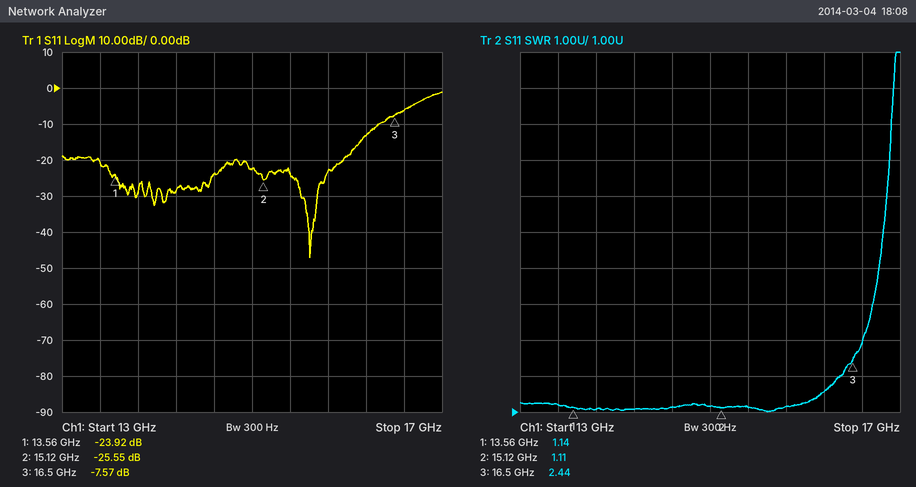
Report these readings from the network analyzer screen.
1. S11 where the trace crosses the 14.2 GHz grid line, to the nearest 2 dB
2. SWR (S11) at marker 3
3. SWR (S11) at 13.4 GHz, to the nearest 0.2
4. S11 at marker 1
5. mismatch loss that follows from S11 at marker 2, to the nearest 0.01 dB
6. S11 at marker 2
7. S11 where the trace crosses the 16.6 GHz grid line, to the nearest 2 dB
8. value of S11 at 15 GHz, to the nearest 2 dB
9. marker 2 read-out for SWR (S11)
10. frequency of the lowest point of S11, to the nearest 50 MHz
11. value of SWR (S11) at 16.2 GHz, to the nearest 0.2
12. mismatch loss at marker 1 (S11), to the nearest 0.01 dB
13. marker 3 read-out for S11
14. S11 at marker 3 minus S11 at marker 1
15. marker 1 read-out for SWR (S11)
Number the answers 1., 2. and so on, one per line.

1. -28 dB
2. 2.44
3. 1.2
4. -23.92 dB
5. 0.01 dB
6. -25.55 dB
7. -6 dB
8. -22 dB
9. 1.11
10. 15.60 GHz
11. 1.6
12. 0.02 dB
13. -7.57 dB
14. 16.35 dB
15. 1.14
